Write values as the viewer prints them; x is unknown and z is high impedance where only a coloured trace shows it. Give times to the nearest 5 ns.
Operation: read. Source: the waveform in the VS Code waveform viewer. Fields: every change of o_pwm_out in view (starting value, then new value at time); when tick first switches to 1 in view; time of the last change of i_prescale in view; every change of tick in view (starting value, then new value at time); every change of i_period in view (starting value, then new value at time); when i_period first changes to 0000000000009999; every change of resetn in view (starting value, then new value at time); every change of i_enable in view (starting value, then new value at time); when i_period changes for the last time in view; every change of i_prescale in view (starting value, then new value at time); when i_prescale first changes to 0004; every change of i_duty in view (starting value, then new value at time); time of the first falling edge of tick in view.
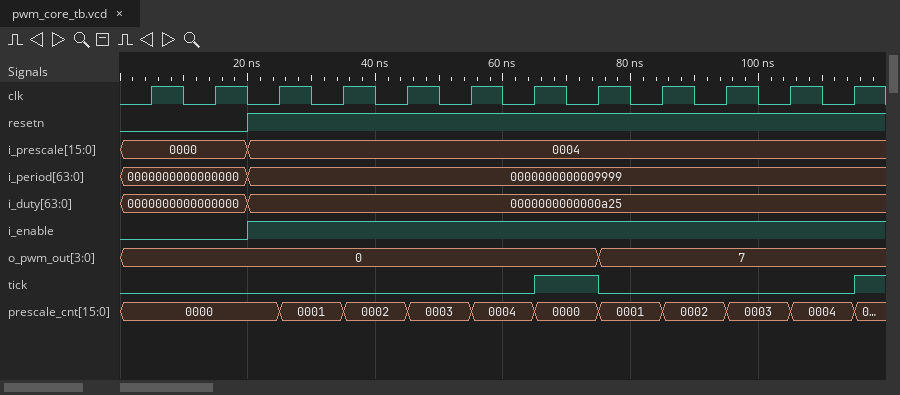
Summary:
0, 7 at 75 ns
65 ns
20 ns
0, 1 at 65 ns, 0 at 75 ns, 1 at 115 ns
0000000000000000, 0000000000009999 at 20 ns
20 ns
0, 1 at 20 ns
0, 1 at 20 ns
20 ns
0000, 0004 at 20 ns
20 ns
0000000000000000, 0000000000000a25 at 20 ns
75 ns
